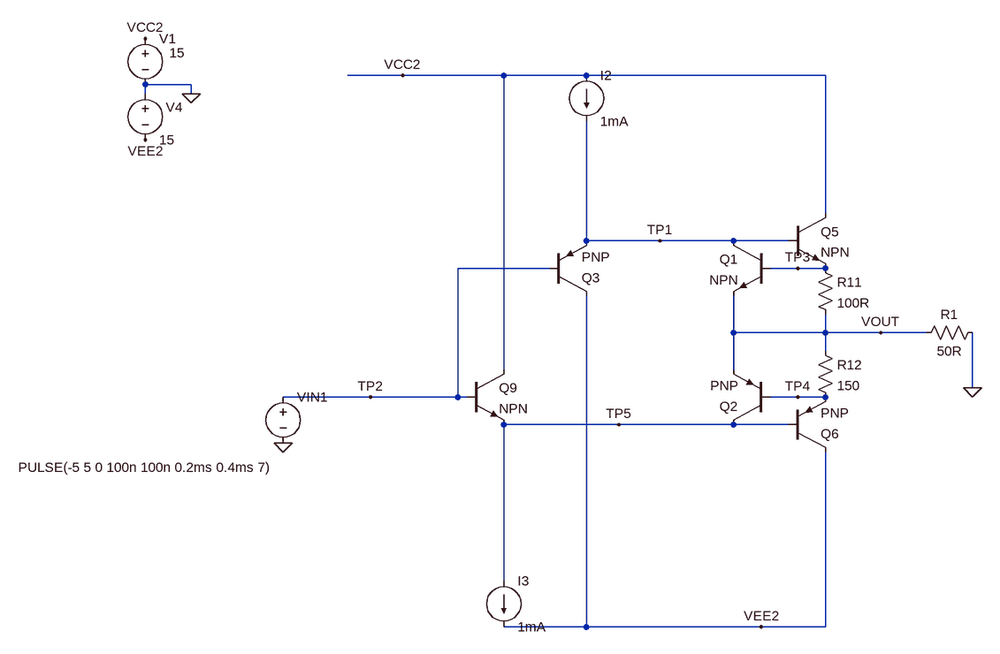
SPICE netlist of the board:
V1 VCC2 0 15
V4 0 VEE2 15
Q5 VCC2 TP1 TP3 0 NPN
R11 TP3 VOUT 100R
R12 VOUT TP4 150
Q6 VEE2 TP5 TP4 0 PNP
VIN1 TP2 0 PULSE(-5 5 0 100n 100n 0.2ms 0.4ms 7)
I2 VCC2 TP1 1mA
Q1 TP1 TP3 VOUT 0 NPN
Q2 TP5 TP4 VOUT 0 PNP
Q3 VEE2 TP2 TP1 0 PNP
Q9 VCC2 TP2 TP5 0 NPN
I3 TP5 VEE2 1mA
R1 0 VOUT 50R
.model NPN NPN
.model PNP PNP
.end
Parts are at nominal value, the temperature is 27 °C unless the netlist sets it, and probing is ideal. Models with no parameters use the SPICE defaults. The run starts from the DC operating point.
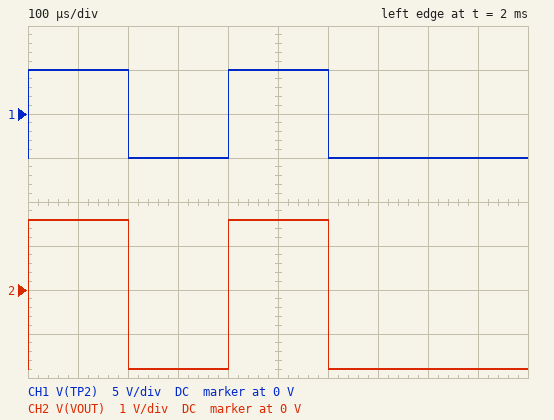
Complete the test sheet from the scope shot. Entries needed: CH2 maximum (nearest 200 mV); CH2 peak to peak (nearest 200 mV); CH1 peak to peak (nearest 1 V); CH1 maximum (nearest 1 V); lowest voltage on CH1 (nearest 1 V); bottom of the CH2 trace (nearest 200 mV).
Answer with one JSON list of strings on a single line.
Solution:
["1.6 V", "3.4 V", "10 V", "5 V", "-5 V", "-1.8 V"]
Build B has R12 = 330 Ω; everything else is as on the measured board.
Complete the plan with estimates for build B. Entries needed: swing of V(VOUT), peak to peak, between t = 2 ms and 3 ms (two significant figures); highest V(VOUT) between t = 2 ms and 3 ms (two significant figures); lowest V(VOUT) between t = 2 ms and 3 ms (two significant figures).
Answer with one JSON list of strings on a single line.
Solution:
["2.8 V", "1.1 V", "-1.7 V"]
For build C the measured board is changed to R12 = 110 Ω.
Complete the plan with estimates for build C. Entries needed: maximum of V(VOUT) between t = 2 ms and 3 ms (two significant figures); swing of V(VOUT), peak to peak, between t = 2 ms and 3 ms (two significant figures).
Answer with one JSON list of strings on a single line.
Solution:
["1.8 V", "3.6 V"]
